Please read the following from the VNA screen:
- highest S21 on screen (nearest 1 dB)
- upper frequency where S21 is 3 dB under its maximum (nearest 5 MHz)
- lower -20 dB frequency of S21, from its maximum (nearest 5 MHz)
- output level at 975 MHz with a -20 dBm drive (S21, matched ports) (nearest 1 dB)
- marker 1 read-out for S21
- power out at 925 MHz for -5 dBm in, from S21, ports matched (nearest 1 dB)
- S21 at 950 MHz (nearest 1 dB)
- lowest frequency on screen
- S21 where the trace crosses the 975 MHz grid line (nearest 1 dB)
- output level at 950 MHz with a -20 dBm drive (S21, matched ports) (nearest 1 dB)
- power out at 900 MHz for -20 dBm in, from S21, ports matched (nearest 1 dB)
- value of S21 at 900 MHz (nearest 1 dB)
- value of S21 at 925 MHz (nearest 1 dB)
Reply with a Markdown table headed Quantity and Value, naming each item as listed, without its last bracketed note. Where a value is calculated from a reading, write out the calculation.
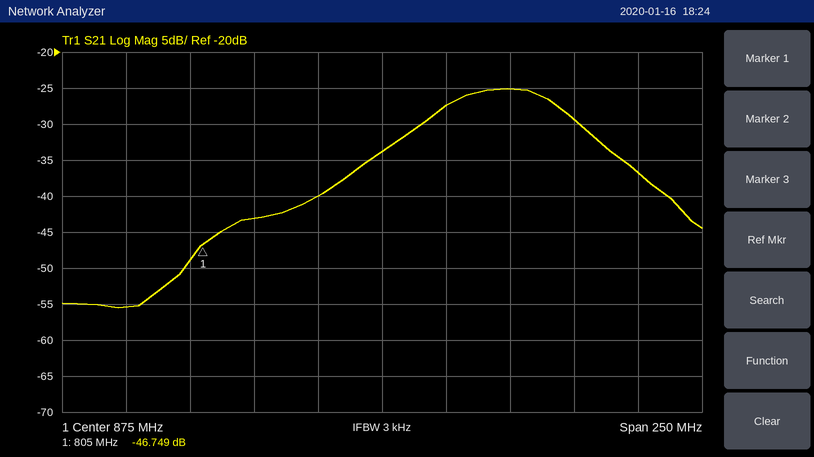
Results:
| Quantity | Value |
|---|---|
| highest S21 on screen | -25 dB |
| upper frequency where S21 is 3 dB under its maximum | 945 MHz |
| lower -20 dB frequency of S21, from its maximum | 810 MHz |
| output level at 975 MHz with a -20 dBm drive (S21, matched ports) | -20 dBm + (-37 dB) = -57 dBm |
| marker 1 read-out for S21 | -46.749 dB |
| power out at 925 MHz for -5 dBm in, from S21, ports matched | -5 dBm + (-25 dB) = -30 dBm |
| S21 at 950 MHz | -29 dB |
| lowest frequency on screen | 750 MHz |
| S21 where the trace crosses the 975 MHz grid line | -37 dB |
| output level at 950 MHz with a -20 dBm drive (S21, matched ports) | -20 dBm + (-29 dB) = -49 dBm |
| power out at 900 MHz for -20 dBm in, from S21, ports matched | -20 dBm + (-27 dB) = -47 dBm |
| value of S21 at 900 MHz | -27 dB |
| value of S21 at 925 MHz | -25 dB |
